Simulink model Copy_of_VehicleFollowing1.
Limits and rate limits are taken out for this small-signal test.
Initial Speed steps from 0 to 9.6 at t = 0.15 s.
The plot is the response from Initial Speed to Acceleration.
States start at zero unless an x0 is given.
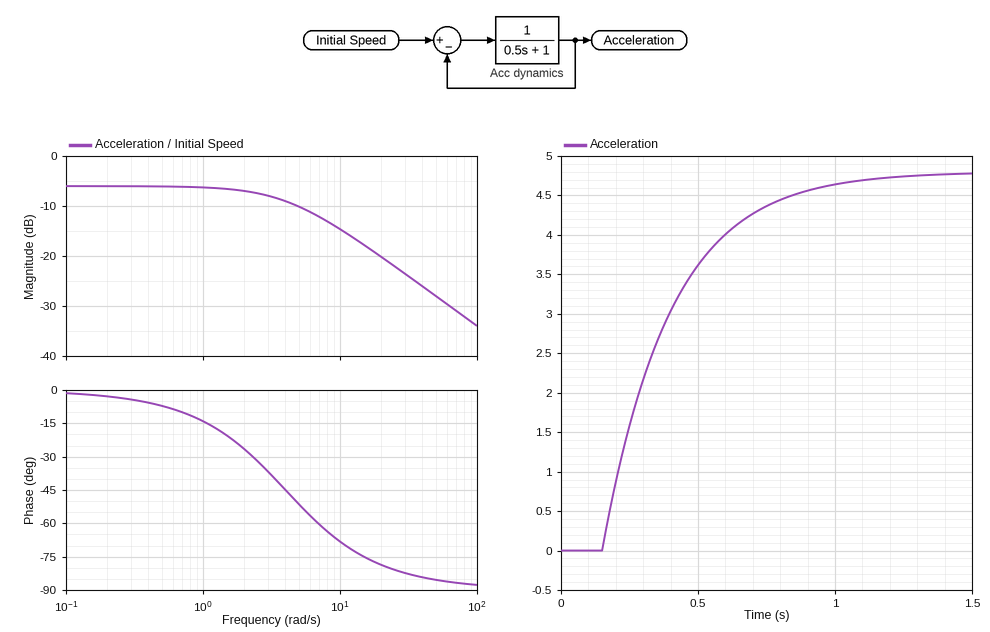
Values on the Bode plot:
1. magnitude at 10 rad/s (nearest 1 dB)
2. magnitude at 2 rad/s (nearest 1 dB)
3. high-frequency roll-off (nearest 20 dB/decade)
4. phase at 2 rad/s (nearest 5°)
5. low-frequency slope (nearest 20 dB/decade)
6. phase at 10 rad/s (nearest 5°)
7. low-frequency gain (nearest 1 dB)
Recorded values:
-15 dB
-7 dB
-20 dB/decade
-25°
0 dB/decade
-70°
-6 dB
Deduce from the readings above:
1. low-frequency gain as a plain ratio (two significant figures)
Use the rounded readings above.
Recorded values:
0.50
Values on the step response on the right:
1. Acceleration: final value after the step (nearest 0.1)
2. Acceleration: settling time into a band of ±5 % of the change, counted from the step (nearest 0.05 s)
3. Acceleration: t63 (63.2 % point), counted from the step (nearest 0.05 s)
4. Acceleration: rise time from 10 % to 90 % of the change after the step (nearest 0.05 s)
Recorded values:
4.8
0.75 s
0.25 s
0.55 s
